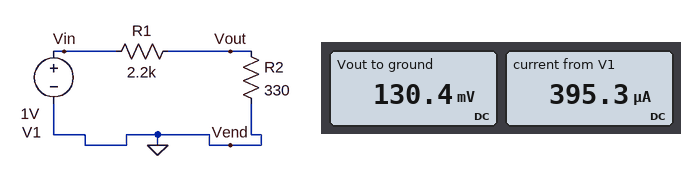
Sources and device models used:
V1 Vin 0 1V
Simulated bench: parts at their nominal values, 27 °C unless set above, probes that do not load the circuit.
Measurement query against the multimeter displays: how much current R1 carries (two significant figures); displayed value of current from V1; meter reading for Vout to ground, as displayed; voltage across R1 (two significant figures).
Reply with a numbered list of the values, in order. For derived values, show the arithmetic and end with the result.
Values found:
1. (1 V - 130.4 mV) / 2.2 kΩ = 400 µA
2. 395.3 µA
3. 130.4 mV
4. 1 V - 130.4 mV = 870 mV
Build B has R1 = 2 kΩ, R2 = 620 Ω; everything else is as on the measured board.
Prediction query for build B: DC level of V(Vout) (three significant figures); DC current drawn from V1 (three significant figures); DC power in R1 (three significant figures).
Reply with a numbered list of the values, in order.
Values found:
1. 237 mV
2. 382 µA
3. 291 µW
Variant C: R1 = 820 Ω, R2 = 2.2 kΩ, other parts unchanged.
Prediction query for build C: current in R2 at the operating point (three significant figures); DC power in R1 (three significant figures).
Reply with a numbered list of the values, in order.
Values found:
1. 331 µA
2. 89.9 µW
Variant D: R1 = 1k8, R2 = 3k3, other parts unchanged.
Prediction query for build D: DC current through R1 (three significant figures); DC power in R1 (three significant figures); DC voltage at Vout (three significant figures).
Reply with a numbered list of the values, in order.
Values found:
1. 196 µA
2. 69.2 µW
3. 647 mV
